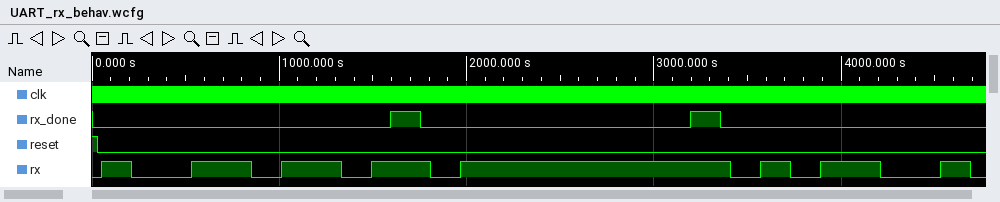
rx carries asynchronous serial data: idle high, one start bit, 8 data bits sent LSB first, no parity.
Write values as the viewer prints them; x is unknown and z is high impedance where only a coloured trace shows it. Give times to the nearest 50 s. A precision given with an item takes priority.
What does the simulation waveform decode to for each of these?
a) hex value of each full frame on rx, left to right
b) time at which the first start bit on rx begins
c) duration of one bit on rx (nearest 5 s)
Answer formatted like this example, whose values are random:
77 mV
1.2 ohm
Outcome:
B6, FF
200 s
160 s
